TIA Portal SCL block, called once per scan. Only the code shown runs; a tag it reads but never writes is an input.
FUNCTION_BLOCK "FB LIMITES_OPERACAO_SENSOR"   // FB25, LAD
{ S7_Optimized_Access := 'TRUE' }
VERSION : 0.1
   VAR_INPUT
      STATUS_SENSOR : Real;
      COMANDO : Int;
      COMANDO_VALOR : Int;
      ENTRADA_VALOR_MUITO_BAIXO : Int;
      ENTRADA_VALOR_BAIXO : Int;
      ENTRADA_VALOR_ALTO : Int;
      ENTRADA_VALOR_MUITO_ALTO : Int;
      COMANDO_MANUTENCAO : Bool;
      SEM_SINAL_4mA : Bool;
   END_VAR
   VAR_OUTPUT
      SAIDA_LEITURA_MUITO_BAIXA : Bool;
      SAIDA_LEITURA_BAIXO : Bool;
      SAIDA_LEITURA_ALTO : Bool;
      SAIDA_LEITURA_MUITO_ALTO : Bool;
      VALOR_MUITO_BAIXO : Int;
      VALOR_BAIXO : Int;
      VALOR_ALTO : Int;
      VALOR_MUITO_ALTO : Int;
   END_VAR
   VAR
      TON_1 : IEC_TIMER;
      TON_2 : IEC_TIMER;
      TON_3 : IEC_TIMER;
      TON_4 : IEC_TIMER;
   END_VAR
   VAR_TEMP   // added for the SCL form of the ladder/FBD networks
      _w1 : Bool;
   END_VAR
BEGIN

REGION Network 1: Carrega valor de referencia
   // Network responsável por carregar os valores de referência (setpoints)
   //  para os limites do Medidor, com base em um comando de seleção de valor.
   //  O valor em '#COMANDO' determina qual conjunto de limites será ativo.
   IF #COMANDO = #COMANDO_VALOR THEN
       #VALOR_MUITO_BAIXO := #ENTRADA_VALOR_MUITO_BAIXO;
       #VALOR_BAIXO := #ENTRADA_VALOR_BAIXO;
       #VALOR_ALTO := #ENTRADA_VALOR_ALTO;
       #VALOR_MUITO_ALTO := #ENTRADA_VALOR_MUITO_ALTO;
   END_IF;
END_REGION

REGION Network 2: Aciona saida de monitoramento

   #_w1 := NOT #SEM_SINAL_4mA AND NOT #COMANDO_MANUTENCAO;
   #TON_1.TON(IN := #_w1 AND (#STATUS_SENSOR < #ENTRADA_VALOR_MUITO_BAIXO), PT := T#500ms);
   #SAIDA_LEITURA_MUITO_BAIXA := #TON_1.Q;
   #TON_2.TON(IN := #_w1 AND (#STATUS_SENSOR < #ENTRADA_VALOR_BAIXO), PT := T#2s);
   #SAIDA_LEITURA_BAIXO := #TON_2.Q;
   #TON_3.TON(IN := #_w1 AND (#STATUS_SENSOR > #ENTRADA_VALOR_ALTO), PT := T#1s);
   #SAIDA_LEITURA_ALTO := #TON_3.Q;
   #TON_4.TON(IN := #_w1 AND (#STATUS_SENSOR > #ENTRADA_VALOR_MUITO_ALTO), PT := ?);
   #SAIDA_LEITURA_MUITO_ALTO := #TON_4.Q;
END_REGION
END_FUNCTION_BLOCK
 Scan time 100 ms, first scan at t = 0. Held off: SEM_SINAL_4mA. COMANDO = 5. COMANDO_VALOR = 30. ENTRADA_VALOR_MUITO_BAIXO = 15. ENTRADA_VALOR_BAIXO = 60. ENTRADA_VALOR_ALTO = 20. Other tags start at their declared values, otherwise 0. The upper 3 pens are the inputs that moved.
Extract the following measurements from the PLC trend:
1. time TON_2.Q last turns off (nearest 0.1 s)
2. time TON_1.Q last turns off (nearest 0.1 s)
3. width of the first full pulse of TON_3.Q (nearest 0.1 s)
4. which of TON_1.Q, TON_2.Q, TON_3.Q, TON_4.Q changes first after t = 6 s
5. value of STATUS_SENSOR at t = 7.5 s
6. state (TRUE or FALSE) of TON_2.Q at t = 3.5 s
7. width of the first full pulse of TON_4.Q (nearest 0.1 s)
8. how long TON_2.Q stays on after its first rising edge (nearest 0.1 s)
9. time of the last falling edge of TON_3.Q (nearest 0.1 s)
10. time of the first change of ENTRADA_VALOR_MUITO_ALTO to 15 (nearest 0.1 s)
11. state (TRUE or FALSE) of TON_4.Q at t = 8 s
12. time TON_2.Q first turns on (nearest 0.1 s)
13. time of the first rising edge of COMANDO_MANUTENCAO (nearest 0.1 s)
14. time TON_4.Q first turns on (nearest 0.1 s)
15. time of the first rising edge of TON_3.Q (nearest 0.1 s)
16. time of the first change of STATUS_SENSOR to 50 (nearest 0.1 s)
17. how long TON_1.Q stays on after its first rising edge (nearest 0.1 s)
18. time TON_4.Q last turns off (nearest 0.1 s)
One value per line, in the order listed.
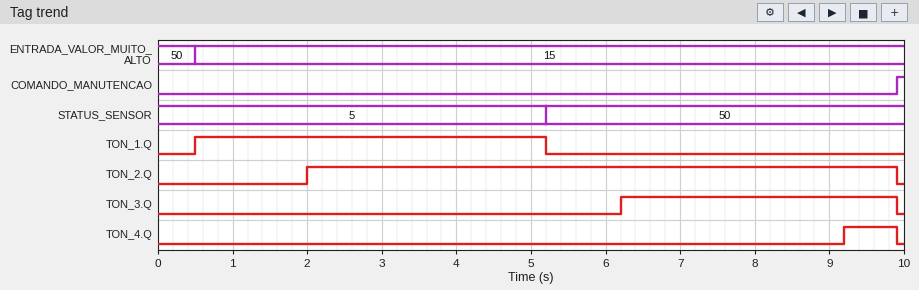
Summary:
9.9 s
5.2 s
3.7 s
TON_3.Q
50
TRUE
0.7 s
7.9 s
9.9 s
0.5 s
FALSE
2.0 s
9.9 s
9.2 s
6.2 s
5.2 s
4.7 s
9.9 s
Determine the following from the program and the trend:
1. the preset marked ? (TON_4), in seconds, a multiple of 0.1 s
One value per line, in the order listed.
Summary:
4.0 s
